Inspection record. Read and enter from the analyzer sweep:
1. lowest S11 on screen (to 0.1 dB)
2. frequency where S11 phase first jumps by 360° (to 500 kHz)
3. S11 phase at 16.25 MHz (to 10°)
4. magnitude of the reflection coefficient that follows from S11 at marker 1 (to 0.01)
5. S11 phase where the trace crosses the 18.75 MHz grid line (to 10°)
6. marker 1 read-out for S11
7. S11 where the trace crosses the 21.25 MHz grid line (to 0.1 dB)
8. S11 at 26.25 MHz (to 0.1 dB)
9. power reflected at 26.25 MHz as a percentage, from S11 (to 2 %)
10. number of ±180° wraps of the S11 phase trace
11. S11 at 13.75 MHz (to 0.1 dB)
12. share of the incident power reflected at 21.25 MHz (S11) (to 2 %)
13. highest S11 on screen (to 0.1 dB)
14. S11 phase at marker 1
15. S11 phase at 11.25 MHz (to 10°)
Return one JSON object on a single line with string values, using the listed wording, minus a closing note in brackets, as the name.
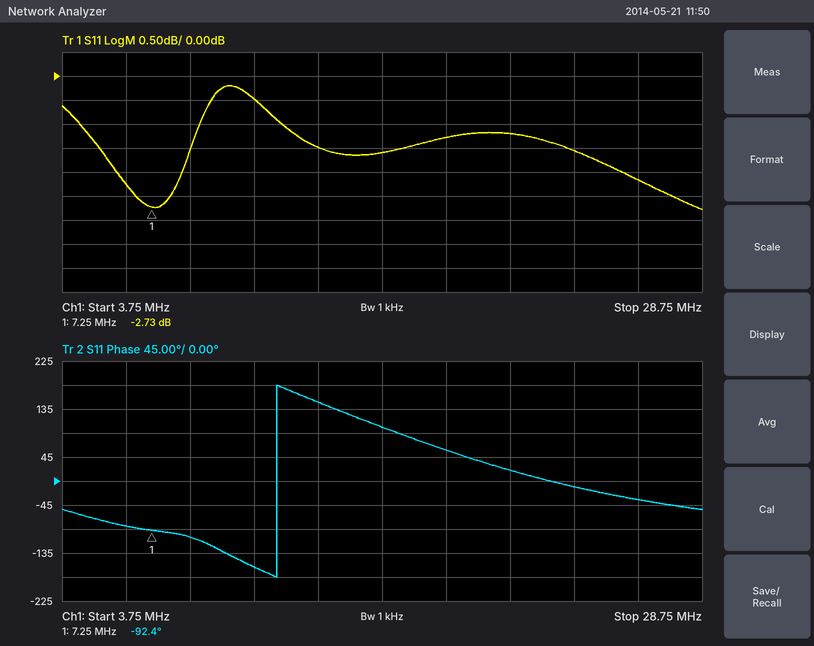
{"lowest S11 on screen": "-2.8 dB", "frequency where S11 phase first jumps by 360°": "12.0 MHz", "S11 phase at 16.25 MHz": "100°", "magnitude of the reflection coefficient that follows from S11 at marker 1": "0.73", "S11 phase where the trace crosses the 18.75 MHz grid line": "60°", "marker 1 read-out for S11": "-2.73 dB", "S11 where the trace crosses the 21.25 MHz grid line": "-1.2 dB", "S11 at 26.25 MHz": "-2.2 dB", "power reflected at 26.25 MHz as a percentage, from S11": "60 %", "number of ±180° wraps of the S11 phase trace": "1", "S11 at 13.75 MHz": "-1.5 dB", "share of the incident power reflected at 21.25 MHz (S11)": "76 %", "highest S11 on screen": "-0.2 dB", "S11 phase at marker 1": "-92.4°", "S11 phase at 11.25 MHz": "-160°"}
